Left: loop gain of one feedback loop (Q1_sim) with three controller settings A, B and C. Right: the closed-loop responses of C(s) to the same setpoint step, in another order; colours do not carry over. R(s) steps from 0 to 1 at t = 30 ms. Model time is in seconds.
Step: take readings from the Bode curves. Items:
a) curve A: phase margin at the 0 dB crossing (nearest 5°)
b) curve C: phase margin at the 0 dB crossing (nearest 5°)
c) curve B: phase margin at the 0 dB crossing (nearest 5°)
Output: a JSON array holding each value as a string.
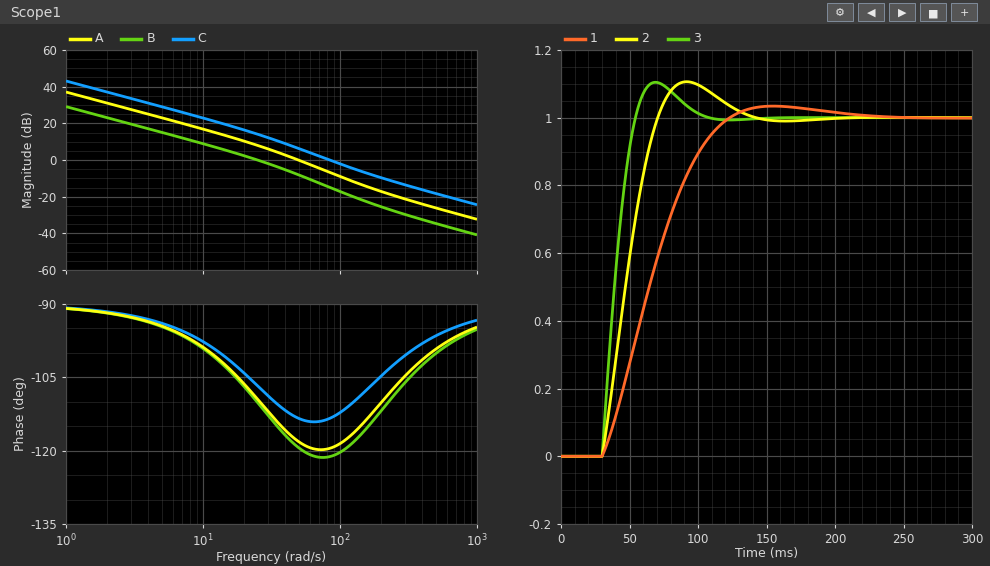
["60°", "65°", "70°"]
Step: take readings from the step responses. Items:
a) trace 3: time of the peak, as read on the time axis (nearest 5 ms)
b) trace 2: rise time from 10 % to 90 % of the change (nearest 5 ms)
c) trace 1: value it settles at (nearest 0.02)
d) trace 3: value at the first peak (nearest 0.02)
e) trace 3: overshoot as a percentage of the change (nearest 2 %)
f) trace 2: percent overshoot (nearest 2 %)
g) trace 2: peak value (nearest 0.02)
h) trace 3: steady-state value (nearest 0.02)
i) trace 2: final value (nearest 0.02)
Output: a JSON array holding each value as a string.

["70 ms", "30 ms", "1.00", "1.10", "10 %", "10 %", "1.10", "1.00", "1.00"]
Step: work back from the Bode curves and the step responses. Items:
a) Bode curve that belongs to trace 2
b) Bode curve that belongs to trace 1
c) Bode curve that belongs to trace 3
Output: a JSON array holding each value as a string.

["A", "B", "C"]
